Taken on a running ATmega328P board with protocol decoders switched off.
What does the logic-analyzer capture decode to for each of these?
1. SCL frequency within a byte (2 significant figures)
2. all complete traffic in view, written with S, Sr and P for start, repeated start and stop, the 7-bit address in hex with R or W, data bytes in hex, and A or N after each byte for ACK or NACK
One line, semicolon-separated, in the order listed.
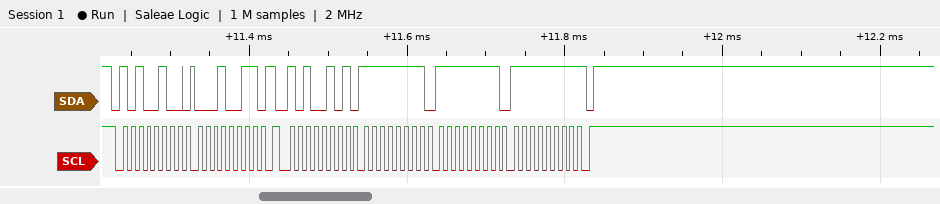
100 kHz; S 52W A 13 A Sr 52R A FF A FF A FF N P
